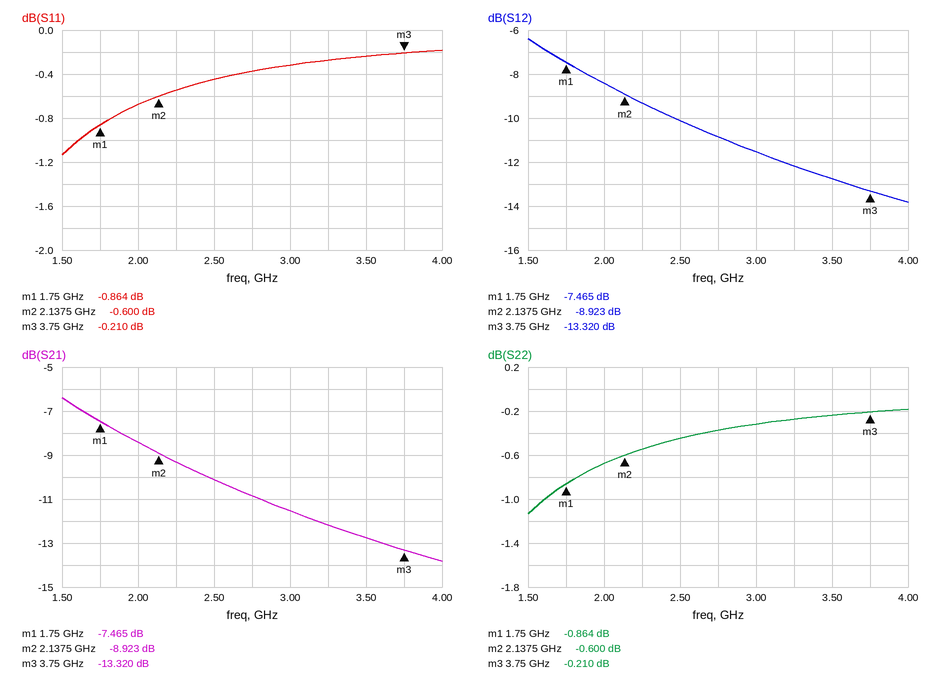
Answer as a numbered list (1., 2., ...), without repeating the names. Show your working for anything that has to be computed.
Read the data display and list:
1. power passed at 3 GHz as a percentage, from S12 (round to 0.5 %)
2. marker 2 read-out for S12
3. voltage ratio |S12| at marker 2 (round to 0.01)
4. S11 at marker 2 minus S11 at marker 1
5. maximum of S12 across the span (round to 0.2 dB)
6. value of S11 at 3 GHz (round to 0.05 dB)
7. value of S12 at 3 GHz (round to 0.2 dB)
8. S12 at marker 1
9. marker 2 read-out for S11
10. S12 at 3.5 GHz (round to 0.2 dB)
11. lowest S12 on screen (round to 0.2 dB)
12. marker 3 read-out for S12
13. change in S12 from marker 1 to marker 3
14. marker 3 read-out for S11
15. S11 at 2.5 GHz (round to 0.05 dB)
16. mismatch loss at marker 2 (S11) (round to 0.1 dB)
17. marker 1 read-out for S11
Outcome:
1. 10^(-11.6/10) ≈ 6.92 %, so 7.0 % to the nearest 0.5 %
2. -8.923 dB
3. 10^(-8.923/20) ≈ 0.36
4. -0.6 − (-0.864) = 0.264 dB
5. -6.4 dB
6. -0.30 dB
7. -11.6 dB
8. -7.465 dB
9. -0.600 dB
10. -12.8 dB
11. -13.8 dB
12. -13.320 dB
13. -13.32 − (-7.465) = -5.855 dB
14. -0.210 dB
15. -0.45 dB
16. −10 log10(1 − 10^(-0.6/10)) ≈ 8.9 dB
17. -0.864 dB
